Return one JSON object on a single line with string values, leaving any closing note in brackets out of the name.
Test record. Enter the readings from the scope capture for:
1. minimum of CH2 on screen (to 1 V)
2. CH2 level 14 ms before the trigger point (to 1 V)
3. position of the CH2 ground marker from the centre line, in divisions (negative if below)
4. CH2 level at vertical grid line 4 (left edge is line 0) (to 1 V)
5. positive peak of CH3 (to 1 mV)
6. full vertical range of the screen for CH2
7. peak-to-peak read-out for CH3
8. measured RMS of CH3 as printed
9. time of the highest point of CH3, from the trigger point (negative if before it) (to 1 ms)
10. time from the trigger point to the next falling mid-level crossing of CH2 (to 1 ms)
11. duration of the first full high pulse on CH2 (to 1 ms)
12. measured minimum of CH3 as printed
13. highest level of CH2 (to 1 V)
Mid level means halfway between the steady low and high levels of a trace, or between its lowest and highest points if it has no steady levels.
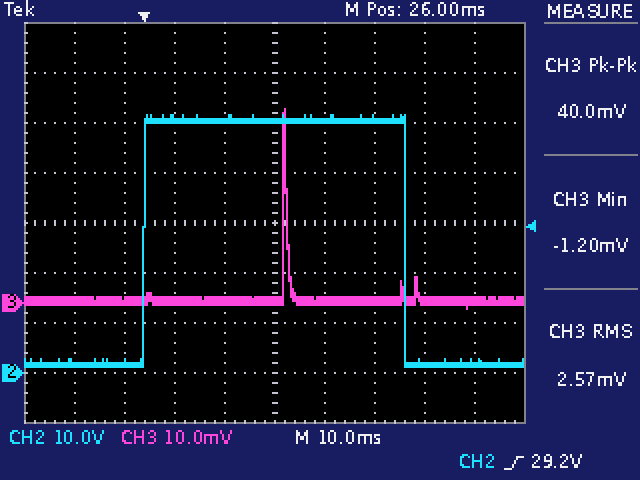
{"minimum of CH2 on screen": "1 V", "CH2 level 14 ms before the trigger point": "2 V", "position of the CH2 ground marker from the centre line, in divisions": "-3.0 div", "CH2 level at vertical grid line 4 (left edge is line 0)": "50 V", "positive peak of CH3": "39 mV", "full vertical range of the screen for CH2": "80 V", "peak-to-peak read-out for CH3": "40.0 mV", "measured RMS of CH3 as printed": "2.57 mV", "time of the highest point of CH3, from the trigger point (negative if before it)": "+28 ms", "time from the trigger point to the next falling mid-level crossing of CH2": "52 ms", "duration of the first full high pulse on CH2": "52 ms", "measured minimum of CH3 as printed": "-1.20 mV", "highest level of CH2": "52 V"}
